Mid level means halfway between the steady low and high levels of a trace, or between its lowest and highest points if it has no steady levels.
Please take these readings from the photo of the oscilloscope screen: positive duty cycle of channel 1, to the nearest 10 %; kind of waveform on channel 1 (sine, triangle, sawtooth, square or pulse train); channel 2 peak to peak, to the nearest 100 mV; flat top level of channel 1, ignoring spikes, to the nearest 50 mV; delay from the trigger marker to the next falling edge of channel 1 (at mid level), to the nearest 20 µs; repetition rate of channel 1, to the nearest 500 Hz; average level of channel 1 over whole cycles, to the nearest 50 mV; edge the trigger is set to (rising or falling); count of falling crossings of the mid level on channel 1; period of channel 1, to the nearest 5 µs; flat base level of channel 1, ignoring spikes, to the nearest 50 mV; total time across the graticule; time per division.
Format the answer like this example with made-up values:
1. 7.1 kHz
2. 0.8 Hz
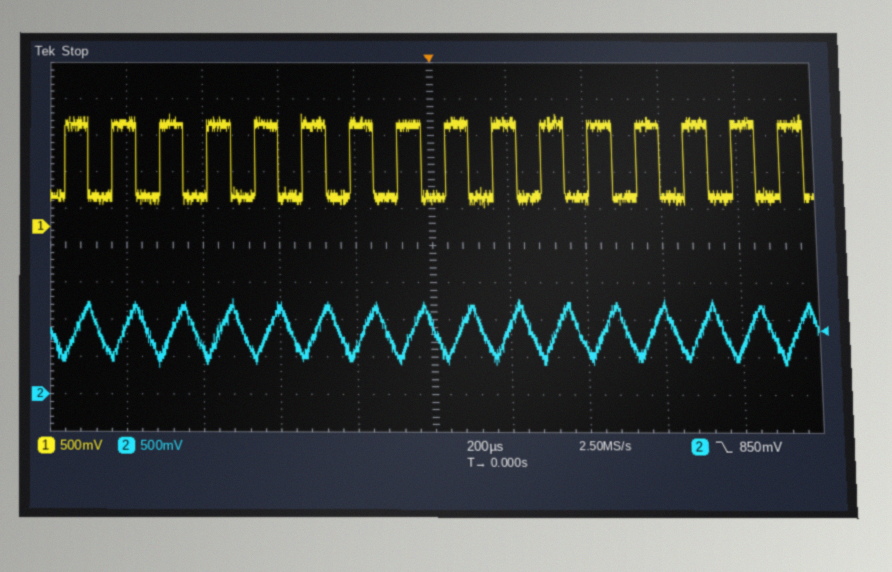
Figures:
1. 50 %
2. square
3. 900 mV
4. 1.40 V
5. 100 µs
6. 8.0 kHz
7. 900 mV
8. falling
9. 16
10. 125 µs
11. 400 mV
12. 2 ms
13. 200 µs
